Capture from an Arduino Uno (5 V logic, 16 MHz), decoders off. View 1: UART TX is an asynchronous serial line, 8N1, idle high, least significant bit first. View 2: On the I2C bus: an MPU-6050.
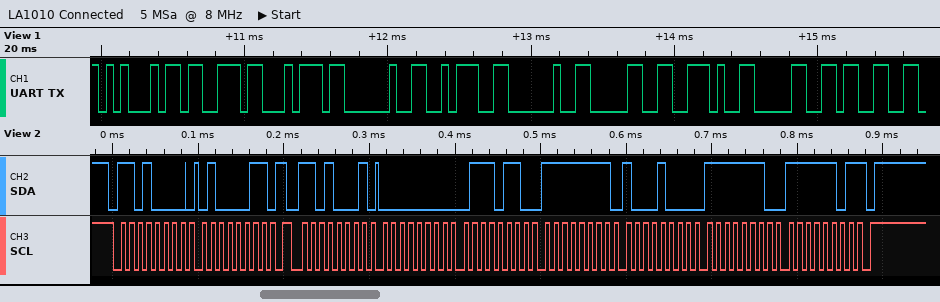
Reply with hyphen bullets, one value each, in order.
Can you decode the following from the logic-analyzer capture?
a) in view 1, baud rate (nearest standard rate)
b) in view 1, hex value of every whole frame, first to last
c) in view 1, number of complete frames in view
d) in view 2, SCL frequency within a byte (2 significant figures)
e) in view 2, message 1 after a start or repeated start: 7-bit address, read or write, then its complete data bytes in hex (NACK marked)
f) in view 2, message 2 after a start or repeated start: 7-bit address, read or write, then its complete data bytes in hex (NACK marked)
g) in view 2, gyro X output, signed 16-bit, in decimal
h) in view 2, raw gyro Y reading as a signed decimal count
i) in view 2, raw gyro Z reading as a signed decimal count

- 19200 baud
- 45 73 74 20 3A 20 30 2E 30 33
- 10
- 100 kHz
- 0x68 write: 43
- 0x68 read: 00 76 FF 88 FE FD NACK
- 118
- -120
- -259
